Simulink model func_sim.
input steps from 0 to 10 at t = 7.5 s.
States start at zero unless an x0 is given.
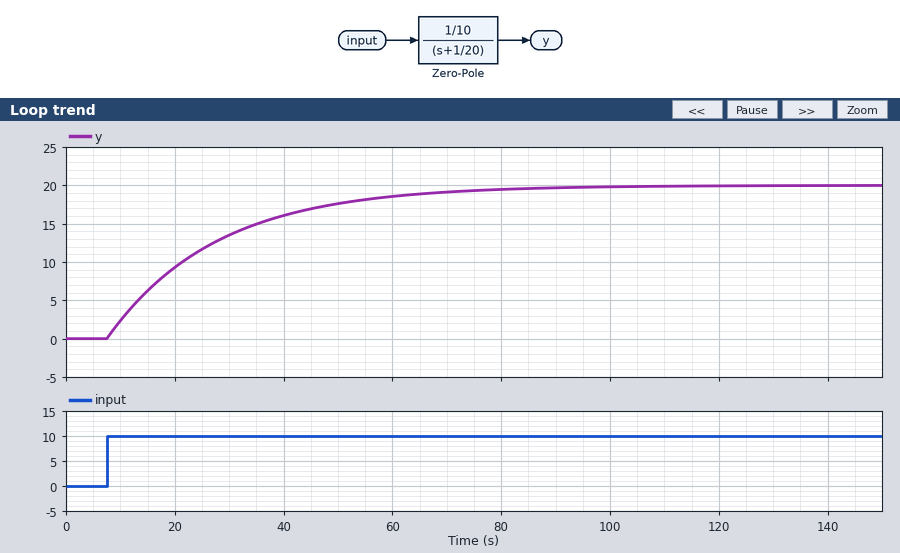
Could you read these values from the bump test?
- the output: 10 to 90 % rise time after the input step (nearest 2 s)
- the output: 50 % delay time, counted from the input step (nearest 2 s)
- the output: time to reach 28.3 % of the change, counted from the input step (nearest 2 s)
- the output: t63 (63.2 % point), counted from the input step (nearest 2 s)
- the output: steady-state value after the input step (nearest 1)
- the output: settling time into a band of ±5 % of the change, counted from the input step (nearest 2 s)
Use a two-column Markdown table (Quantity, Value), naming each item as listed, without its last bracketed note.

| Quantity | Value |
|---|---|
| the output: 10 to 90 % rise time after the input step | 44 s |
| the output: 50 % delay time, counted from the input step | 14 s |
| the output: time to reach 28.3 % of the change, counted from the input step | 6 s |
| the output: t63 (63.2 % point), counted from the input step | 20 s |
| the output: steady-state value after the input step | 20 |
| the output: settling time into a band of ±5 % of the change, counted from the input step | 60 s |
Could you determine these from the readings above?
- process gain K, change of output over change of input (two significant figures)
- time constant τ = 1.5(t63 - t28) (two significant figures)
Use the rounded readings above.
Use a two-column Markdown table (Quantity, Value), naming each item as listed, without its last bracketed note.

| Quantity | Value |
|---|---|
| process gain K, change of output over change of input | 2.0 |
| time constant τ = 1.5(t63 - t28) | 21 s |
